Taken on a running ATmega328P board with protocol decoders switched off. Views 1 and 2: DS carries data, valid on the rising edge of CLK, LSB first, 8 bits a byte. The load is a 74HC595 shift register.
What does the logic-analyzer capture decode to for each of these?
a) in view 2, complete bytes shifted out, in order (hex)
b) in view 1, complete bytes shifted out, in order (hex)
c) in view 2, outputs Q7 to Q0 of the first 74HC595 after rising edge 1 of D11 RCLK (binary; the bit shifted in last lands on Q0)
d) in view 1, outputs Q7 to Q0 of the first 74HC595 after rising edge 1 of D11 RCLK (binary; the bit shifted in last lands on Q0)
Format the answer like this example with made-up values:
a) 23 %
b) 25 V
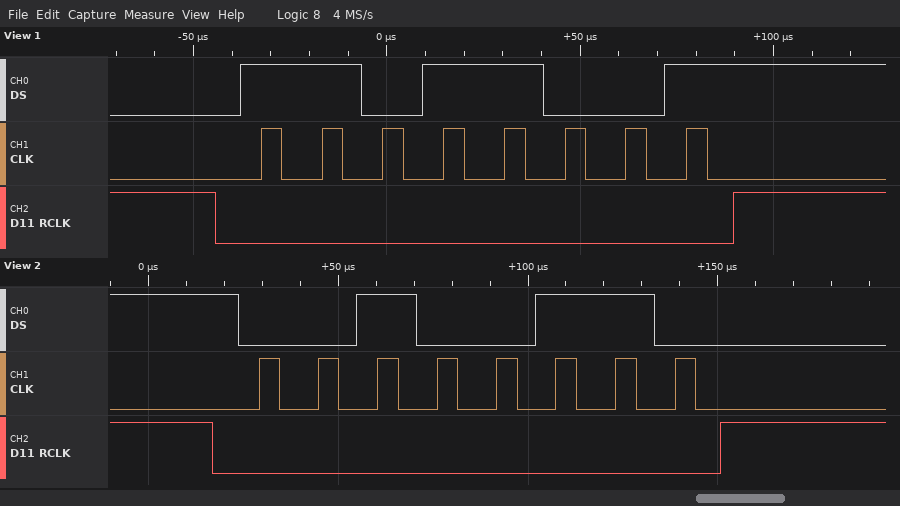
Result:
a) 0x64
b) 9B
c) 00100110
d) 11011001
